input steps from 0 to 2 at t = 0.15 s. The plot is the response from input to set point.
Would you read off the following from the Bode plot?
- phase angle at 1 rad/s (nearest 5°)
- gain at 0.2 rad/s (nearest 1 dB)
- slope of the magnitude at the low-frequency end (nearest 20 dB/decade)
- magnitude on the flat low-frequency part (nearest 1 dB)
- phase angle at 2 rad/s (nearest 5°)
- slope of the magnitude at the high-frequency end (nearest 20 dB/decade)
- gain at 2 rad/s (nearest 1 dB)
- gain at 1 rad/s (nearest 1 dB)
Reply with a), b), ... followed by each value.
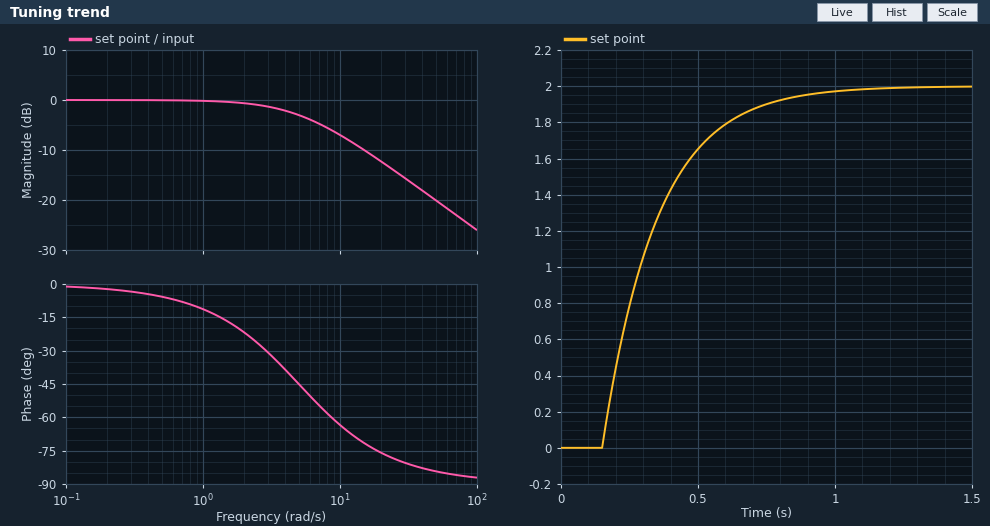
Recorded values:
a) -10°
b) 0 dB
c) 0 dB/decade
d) 0 dB
e) -20°
f) -20 dB/decade
g) -1 dB
h) 0 dB
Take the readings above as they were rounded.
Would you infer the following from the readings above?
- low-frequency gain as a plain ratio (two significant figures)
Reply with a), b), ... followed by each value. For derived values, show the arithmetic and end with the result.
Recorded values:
a) 10^(0 / 20) = 1.0
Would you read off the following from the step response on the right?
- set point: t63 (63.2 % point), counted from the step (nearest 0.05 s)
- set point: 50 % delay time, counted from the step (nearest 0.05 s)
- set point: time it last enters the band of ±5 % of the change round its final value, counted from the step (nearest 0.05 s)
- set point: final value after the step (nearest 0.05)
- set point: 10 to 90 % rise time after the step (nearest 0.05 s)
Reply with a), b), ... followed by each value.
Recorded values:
a) 0.20 s
b) 0.15 s
c) 0.60 s
d) 2.00
e) 0.45 s
